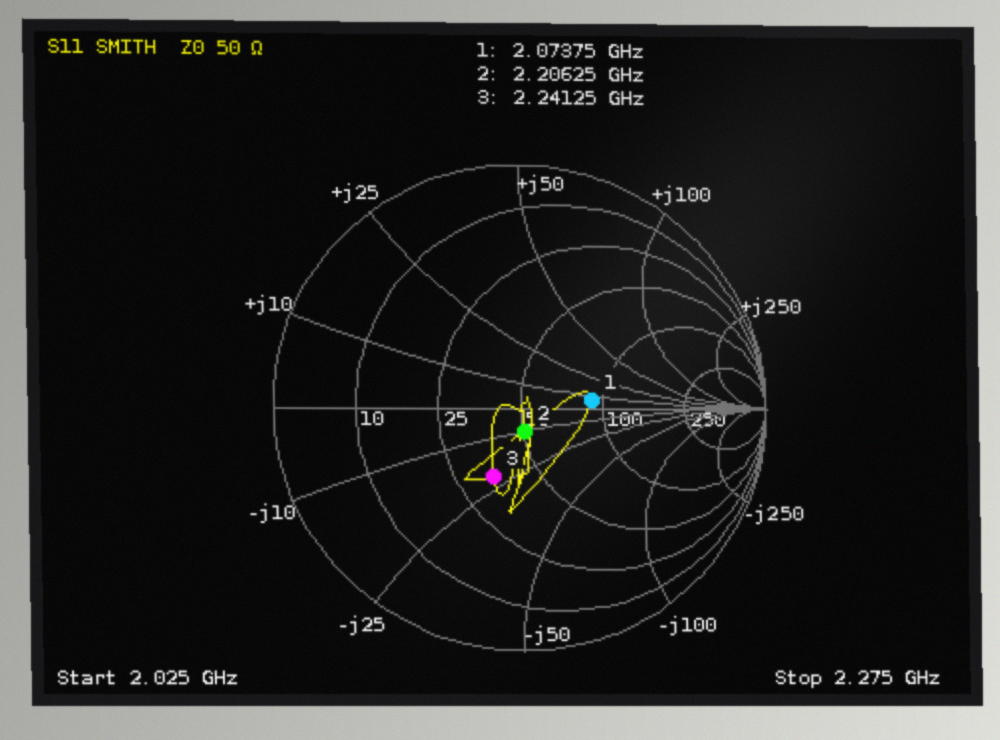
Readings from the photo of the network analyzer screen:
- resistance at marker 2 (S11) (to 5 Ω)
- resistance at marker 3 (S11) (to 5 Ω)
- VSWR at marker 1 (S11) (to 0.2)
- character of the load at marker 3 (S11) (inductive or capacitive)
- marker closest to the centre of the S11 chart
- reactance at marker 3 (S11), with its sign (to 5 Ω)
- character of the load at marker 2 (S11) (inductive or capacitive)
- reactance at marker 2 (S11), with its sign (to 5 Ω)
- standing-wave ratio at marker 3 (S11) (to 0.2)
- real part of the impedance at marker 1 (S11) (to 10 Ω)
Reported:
50 Ω
35 Ω
1.8
capacitive
marker 2
-20 Ω
capacitive
-10 Ω
1.8
90 Ω
